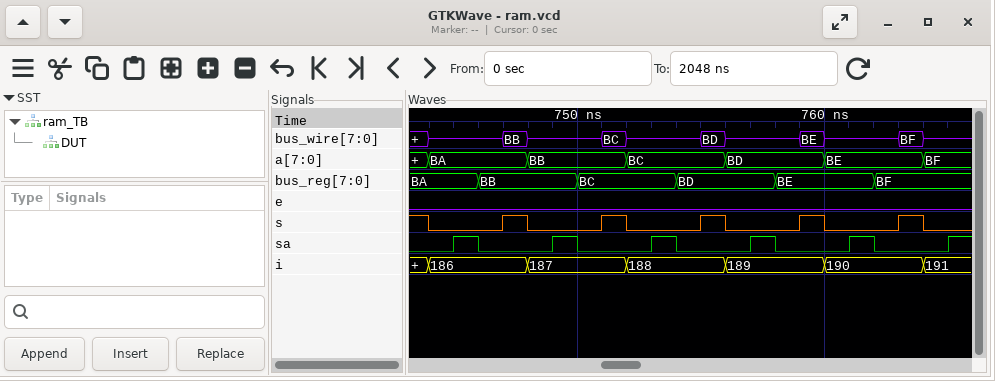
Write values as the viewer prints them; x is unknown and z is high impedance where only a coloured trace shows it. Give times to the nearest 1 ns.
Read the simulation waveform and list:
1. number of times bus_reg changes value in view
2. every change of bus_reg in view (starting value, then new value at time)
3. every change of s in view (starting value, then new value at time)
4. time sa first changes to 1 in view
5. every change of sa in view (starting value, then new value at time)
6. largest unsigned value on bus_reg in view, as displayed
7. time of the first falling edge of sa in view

5
BA, BB at 746 ns, BC at 750 ns, BD at 754 ns, BE at 758 ns, BF at 762 ns
1, 0 at 744 ns, 1 at 747 ns, 0 at 748 ns, 1 at 751 ns, 0 at 752 ns, 1 at 755 ns, 0 at 756 ns, 1 at 759 ns, 0 at 760 ns, 1 at 763 ns, 0 at 764 ns
745 ns
0, 1 at 745 ns, 0 at 746 ns, 1 at 749 ns, 0 at 750 ns, 1 at 753 ns, 0 at 754 ns, 1 at 757 ns, 0 at 758 ns, 1 at 761 ns, 0 at 762 ns, 1 at 765 ns
BF
746 ns
